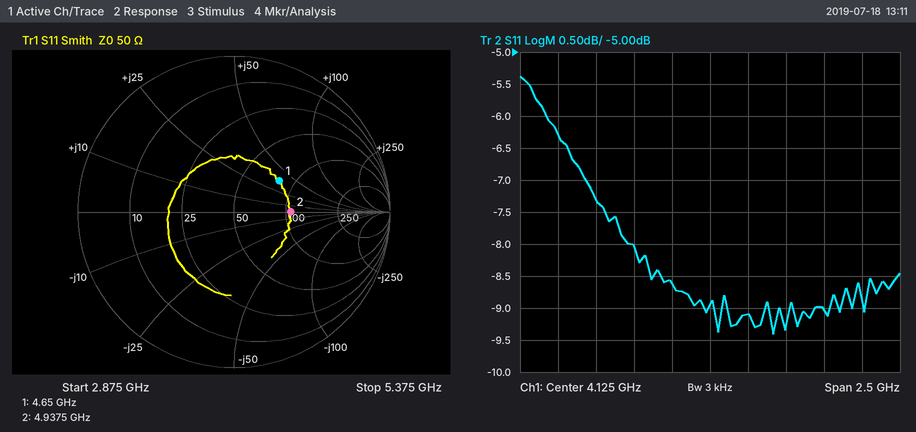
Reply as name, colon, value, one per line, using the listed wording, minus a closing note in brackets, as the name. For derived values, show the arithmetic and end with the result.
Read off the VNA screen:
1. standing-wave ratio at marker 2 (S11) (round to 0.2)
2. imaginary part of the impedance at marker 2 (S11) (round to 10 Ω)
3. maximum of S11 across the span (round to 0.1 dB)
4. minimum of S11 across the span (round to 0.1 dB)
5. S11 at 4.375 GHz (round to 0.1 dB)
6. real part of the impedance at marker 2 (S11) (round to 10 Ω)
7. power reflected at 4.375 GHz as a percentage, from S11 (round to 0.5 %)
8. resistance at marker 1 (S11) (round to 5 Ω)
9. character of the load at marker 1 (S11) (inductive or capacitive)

standing-wave ratio at marker 2 (S11): 2.2
imaginary part of the impedance at marker 2 (S11): 0 Ω
maximum of S11 across the span: -5.4 dB
minimum of S11 across the span: -9.4 dB
S11 at 4.375 GHz: -9.1 dB
real part of the impedance at marker 2 (S11): 110 Ω
power reflected at 4.375 GHz as a percentage, from S11: 10^(-9.1/10) ≈ 12.3 %, so 12.5 % to the nearest 0.5 %
resistance at marker 1 (S11): 80 Ω
character of the load at marker 1 (S11): inductive
